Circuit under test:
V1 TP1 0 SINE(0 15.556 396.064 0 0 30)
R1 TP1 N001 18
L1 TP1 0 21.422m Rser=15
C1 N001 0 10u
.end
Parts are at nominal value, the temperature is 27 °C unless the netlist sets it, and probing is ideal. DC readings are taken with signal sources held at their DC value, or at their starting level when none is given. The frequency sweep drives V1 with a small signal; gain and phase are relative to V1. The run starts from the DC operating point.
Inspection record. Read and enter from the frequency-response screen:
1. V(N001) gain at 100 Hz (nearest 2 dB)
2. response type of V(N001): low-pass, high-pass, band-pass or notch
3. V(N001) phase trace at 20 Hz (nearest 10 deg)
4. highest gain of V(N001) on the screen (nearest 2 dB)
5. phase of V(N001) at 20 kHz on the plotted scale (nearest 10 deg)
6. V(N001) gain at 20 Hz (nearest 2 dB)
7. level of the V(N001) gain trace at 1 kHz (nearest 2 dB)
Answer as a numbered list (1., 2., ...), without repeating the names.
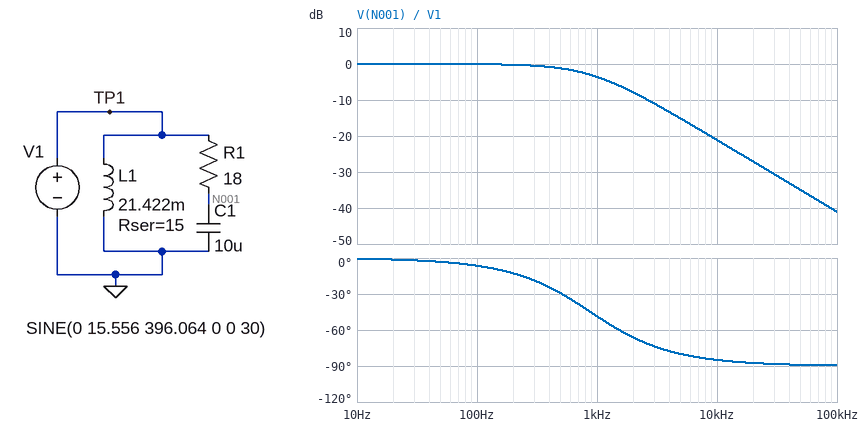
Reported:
1. 0 dB
2. low-pass
3. 0 deg
4. 0 dB
5. -90 deg
6. 0 dB
7. -4 dB
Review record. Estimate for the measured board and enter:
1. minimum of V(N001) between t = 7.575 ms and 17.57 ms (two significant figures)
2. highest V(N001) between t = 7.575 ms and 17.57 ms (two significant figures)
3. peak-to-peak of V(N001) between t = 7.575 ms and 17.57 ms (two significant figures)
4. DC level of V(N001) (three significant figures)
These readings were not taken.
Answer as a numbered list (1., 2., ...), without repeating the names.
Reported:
1. -14 V
2. 14 V
3. 28 V
4. 7.78 V
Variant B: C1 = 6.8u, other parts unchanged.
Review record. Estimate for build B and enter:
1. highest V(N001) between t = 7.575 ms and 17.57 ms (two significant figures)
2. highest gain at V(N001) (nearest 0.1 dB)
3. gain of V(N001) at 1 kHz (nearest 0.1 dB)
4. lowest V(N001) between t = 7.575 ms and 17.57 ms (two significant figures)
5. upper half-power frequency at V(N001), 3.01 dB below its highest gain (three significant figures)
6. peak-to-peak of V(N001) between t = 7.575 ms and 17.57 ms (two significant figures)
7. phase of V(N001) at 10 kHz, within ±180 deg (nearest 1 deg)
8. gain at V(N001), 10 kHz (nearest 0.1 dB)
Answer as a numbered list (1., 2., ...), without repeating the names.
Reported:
1. 15 V
2. 0 dB
3. -2.0 dB
4. -15 V
5. 1.30 kHz
6. 30 V
7. -83 deg
8. -17.8 dB
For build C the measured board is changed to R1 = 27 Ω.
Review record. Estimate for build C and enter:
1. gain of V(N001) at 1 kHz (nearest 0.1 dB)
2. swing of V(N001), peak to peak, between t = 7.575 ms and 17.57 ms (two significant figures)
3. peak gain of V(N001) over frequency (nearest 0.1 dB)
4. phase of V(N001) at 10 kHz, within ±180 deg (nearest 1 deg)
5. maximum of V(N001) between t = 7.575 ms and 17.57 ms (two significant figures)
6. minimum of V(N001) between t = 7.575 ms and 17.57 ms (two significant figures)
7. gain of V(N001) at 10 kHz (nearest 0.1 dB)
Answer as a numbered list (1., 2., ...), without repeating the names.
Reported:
1. -5.9 dB
2. 26 V
3. 0 dB
4. -87 deg
5. 13 V
6. -13 V
7. -24.6 dB
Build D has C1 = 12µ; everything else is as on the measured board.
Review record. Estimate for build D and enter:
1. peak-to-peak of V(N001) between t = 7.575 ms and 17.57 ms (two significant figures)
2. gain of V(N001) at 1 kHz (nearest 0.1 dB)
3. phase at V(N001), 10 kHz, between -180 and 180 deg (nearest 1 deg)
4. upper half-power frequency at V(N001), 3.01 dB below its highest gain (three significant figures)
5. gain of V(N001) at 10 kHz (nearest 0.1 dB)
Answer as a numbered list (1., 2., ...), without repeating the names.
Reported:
1. 27 V
2. -4.5 dB
3. -86 deg
4. 737 Hz
5. -22.7 dB
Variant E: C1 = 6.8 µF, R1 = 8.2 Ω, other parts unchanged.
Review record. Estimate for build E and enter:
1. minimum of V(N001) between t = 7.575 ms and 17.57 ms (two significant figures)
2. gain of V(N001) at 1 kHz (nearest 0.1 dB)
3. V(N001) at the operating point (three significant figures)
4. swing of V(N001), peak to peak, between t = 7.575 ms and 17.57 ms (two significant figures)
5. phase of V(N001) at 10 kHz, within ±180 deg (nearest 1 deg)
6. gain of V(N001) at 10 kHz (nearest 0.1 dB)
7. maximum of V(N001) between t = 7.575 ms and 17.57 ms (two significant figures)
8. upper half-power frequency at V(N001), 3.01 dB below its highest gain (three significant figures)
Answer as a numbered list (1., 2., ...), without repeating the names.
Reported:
1. -15 V
2. -0.5 dB
3. 7.78 V
4. 31 V
5. -74 deg
6. -11.2 dB
7. 15 V
8. 2.85 kHz
